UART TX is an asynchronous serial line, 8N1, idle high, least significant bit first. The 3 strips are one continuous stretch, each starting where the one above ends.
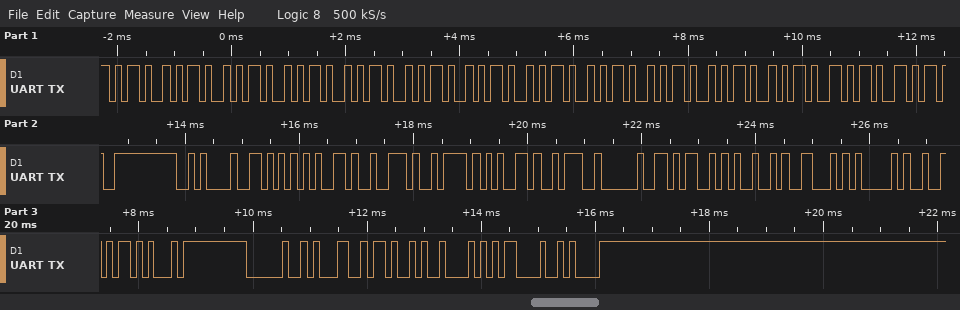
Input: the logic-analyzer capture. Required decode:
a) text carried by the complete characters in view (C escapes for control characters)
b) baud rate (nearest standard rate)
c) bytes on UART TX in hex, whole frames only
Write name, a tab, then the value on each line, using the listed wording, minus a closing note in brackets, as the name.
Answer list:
text carried by the complete characters in view	"--------------\nVerze: MIFARE 1KB\r\n"
baud rate	9600 baud
bytes on UART TX in hex, whole frames only	2D 2D 2D 2D 2D 2D 2D 2D 2D 2D 2D 2D 2D 2D 0A 56 65 72 7A 65 3A 20 4D 49 46 41 52 45 20 31 4B 42 0D 0A
